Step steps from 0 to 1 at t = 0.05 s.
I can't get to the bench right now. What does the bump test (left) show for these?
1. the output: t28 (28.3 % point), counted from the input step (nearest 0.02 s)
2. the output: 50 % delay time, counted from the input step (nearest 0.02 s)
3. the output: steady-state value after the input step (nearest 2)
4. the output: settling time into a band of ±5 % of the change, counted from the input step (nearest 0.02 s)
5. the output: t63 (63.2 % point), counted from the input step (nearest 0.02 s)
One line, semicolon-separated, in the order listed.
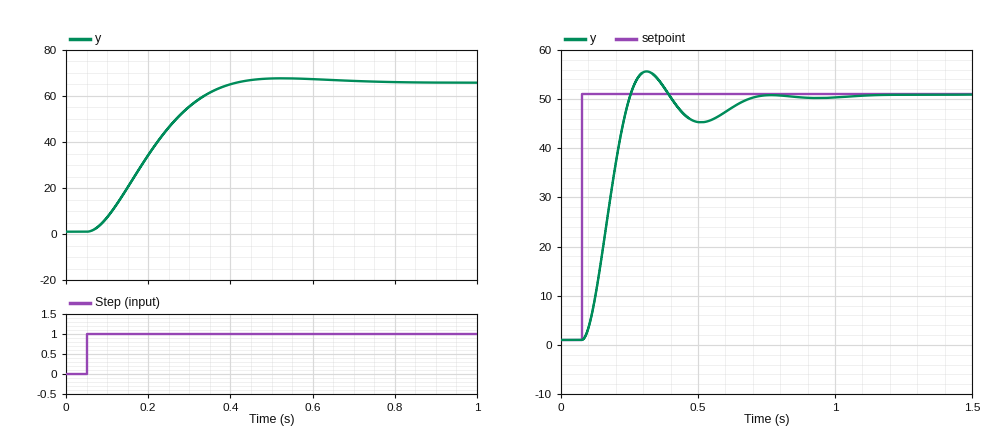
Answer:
0.10 s; 0.14 s; 66; 0.32 s; 0.18 s
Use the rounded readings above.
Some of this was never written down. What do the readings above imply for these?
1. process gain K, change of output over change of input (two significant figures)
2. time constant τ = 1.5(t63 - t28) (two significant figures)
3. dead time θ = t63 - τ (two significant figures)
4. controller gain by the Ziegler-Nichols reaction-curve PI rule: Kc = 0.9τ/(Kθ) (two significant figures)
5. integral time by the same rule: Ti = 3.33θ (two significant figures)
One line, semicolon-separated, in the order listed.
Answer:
66; 0.12 s; 0.060 s; 0.027; 0.20 s
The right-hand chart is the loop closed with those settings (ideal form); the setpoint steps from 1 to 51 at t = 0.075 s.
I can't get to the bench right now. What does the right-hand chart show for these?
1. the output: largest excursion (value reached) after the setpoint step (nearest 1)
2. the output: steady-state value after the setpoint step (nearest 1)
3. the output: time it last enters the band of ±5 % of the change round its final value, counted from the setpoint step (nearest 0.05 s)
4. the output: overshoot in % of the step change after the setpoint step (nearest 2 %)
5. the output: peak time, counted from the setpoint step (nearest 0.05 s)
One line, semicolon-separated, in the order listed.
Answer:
56; 51; 0.55 s; 10 %; 0.25 s
